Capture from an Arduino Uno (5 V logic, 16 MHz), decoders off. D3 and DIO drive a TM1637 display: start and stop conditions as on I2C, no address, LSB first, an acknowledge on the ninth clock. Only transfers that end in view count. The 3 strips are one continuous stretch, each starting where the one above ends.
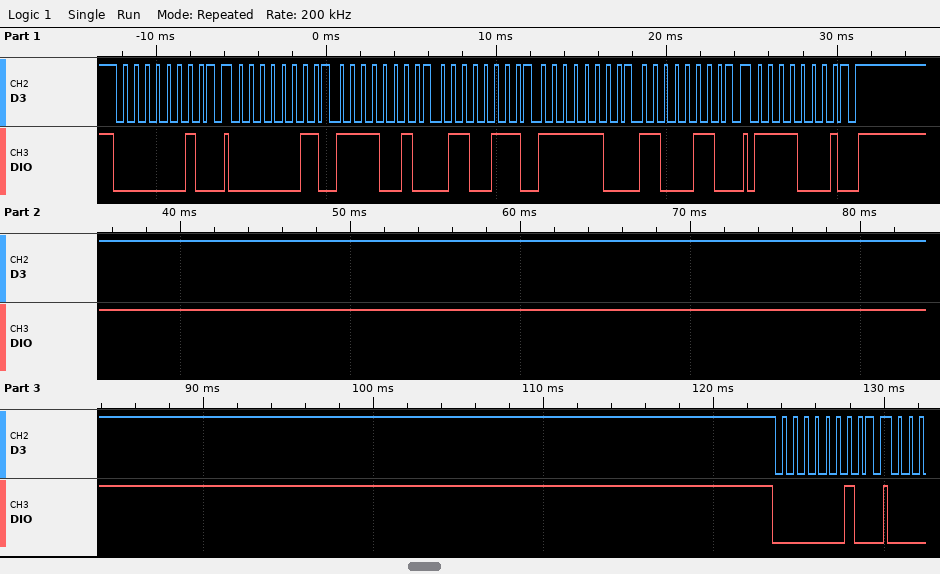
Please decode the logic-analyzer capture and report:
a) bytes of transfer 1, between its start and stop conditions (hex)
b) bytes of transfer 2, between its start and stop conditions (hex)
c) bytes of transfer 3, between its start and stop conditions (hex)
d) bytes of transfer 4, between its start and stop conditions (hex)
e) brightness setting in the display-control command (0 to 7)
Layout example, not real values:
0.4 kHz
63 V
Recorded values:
40
C0 4F E6 3F 63
8F
40
7
